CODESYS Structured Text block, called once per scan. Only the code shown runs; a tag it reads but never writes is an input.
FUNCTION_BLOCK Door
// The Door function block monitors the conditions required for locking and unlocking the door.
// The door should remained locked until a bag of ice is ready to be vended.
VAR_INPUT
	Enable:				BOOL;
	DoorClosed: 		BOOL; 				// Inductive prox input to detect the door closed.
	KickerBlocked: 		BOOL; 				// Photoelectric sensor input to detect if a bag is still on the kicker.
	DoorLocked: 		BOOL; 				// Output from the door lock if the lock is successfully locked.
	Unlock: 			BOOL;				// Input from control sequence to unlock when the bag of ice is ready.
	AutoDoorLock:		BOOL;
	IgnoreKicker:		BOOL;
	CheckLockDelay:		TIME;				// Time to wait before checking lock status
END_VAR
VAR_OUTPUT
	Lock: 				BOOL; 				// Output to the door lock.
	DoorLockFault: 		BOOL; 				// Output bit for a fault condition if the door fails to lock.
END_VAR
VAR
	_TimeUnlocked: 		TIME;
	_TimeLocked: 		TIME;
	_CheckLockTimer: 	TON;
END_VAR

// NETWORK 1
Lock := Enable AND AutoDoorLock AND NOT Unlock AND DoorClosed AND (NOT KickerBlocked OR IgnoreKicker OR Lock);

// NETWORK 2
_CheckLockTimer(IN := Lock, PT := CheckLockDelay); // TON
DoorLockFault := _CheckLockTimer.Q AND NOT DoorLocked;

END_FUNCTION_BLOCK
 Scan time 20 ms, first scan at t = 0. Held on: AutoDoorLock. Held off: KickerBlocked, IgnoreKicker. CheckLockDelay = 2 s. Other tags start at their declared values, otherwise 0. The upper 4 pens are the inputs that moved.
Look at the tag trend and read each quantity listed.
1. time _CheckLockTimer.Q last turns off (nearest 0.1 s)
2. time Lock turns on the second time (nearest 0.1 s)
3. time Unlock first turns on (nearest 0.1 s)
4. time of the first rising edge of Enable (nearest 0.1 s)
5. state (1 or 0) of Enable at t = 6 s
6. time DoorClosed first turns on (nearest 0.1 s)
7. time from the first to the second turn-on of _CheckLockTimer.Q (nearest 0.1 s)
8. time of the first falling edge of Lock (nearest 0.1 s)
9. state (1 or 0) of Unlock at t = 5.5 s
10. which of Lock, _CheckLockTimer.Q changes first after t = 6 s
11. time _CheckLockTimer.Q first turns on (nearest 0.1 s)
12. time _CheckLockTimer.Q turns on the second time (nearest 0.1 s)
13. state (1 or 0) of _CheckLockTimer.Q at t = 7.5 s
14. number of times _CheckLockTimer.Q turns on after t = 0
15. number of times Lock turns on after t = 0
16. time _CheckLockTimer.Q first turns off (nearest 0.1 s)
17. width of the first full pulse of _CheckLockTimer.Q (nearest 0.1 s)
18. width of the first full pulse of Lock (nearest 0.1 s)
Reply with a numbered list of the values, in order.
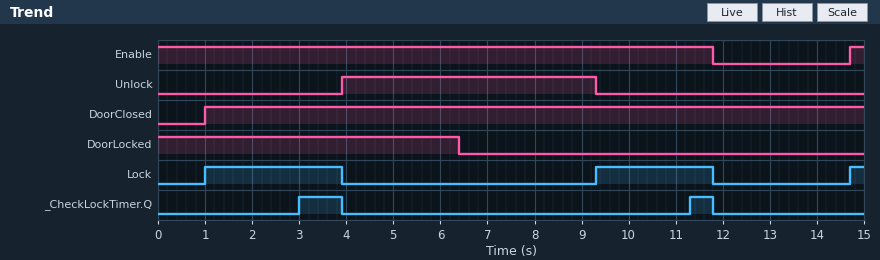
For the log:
1. 11.8 s
2. 9.3 s
3. 3.9 s
4. 14.7 s
5. 1
6. 1.0 s
7. 8.3 s
8. 3.9 s
9. 1
10. Lock
11. 3.0 s
12. 11.3 s
13. 0
14. 2
15. 3
16. 3.9 s
17. 0.9 s
18. 2.9 s
